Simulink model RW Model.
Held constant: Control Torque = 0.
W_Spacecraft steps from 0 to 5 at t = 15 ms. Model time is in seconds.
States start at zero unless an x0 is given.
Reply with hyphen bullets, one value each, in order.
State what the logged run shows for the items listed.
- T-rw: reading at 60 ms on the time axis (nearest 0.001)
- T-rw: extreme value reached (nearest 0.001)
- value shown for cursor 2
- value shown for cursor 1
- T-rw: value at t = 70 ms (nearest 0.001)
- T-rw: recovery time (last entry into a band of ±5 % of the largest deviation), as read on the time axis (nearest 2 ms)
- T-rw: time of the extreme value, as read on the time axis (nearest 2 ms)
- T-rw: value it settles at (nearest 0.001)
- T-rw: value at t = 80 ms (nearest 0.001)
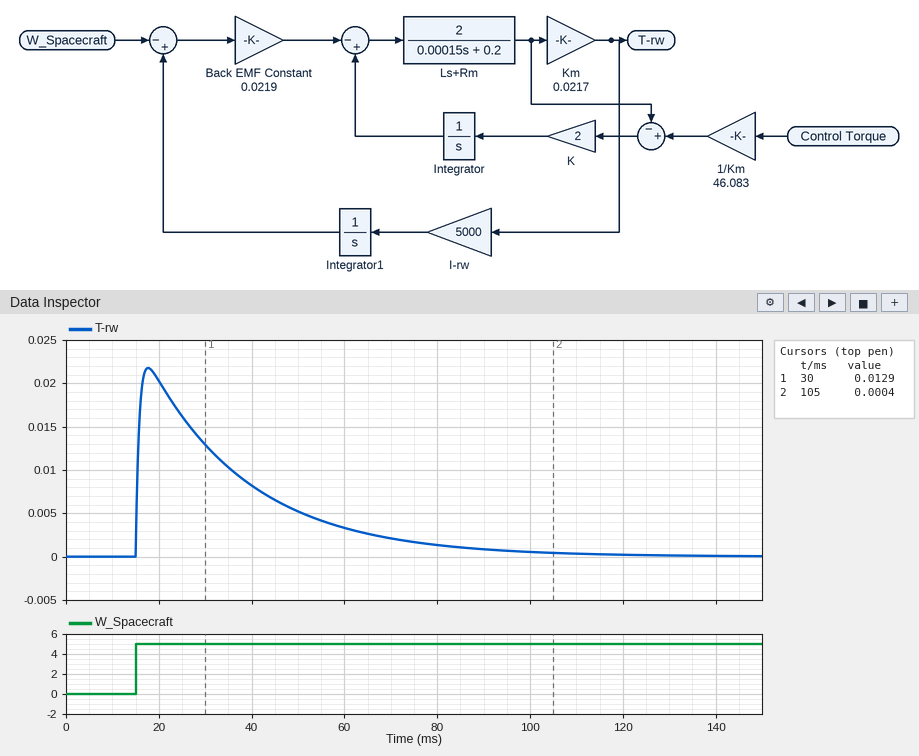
- 0.003
- 0.022
- 0.0004
- 0.0129
- 0.002
- 84 ms
- 18 ms
- 0.000
- 0.001
